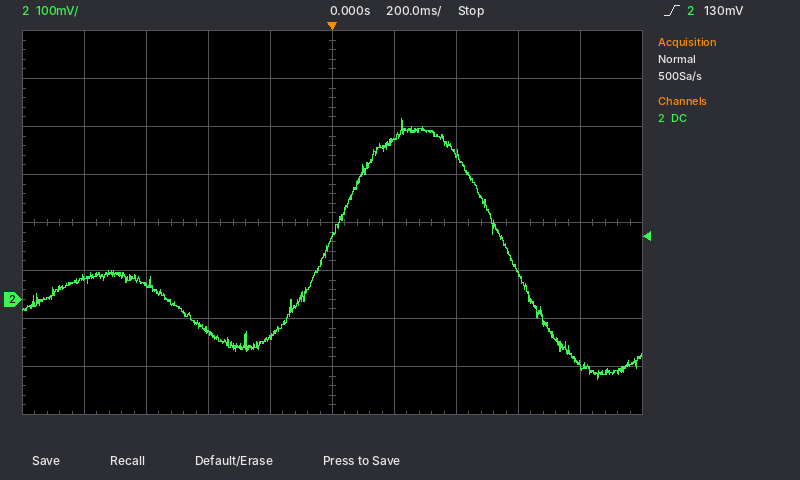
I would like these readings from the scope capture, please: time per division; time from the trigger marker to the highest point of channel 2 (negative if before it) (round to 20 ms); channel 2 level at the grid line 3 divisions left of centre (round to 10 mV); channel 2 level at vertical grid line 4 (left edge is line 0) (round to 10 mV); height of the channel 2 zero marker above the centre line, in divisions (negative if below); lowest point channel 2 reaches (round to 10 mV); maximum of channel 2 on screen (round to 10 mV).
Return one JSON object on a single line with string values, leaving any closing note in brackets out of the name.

{"time per division": "200 ms", "time from the trigger marker to the highest point of channel 2 (negative if before it)": "+220 ms", "channel 2 level at the grid line 3 divisions left of centre": "30 mV", "channel 2 level at vertical grid line 4 (left edge is line 0)": "-80 mV", "height of the channel 2 zero marker above the centre line, in divisions": "-1.6 div", "lowest point channel 2 reaches": "-170 mV", "maximum of channel 2 on screen": "380 mV"}
